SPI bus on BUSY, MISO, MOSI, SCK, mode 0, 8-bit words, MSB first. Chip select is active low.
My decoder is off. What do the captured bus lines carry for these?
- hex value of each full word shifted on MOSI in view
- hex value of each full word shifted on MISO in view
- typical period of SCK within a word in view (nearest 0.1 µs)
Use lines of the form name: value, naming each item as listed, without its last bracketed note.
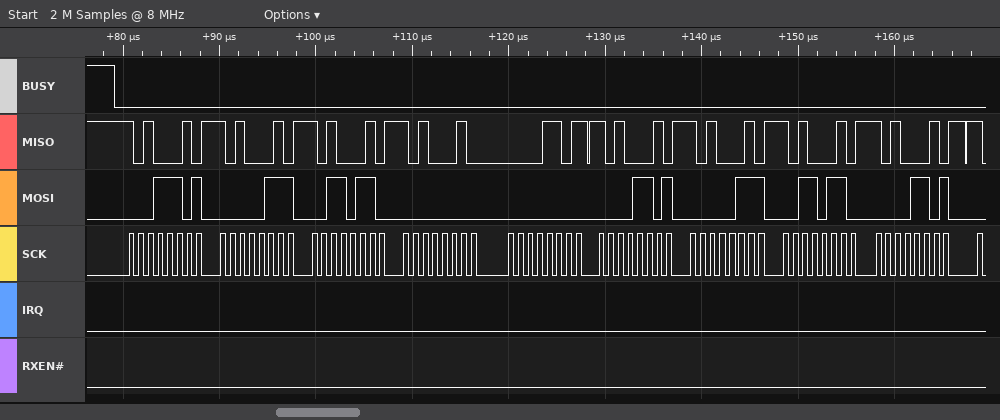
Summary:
hex value of each full word shifted on MOSI in view: 1D, 07, 36, 00, 00, 0D, 07, 36, 0D
hex value of each full word shifted on MISO in view: A2, A2, A2, A2, 0D, A2, A2, A2, A2
typical period of SCK within a word in view: 1 µs
